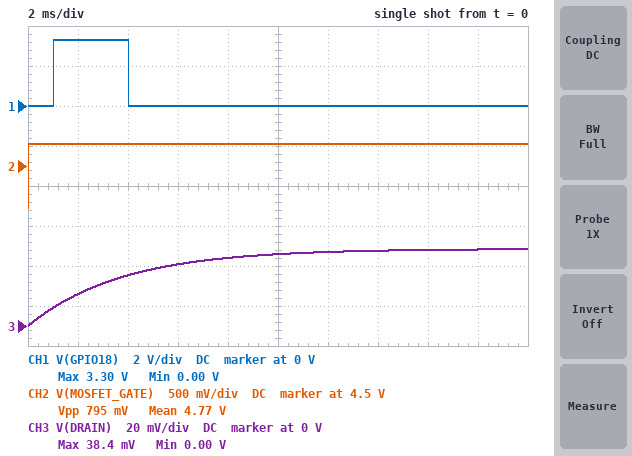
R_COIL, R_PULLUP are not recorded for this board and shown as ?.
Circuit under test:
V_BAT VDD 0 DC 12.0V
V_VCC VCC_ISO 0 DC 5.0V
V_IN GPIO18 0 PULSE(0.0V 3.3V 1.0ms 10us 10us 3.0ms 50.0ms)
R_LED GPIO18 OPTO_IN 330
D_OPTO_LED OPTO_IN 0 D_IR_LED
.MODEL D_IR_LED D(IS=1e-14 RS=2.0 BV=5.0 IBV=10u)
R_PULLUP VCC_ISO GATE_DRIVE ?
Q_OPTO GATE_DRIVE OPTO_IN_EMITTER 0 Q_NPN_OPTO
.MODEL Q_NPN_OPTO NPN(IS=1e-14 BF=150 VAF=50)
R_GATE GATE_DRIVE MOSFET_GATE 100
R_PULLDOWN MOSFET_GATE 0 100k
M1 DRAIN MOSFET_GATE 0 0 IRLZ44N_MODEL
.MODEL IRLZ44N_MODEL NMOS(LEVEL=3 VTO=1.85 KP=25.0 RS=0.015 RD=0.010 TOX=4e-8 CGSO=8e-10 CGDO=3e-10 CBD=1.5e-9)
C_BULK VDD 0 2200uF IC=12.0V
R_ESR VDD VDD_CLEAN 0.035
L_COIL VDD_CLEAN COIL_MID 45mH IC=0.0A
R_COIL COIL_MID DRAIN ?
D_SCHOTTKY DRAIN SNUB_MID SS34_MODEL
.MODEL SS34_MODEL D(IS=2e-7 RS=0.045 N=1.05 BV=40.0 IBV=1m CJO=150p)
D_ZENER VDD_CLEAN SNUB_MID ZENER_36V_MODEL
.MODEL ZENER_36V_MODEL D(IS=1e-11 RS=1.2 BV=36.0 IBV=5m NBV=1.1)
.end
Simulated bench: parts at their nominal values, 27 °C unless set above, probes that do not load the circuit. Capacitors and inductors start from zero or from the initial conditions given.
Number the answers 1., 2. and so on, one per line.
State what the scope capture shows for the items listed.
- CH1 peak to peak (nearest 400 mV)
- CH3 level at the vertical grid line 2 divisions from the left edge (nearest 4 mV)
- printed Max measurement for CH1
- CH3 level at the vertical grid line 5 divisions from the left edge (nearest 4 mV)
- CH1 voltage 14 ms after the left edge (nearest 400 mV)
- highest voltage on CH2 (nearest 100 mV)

1. 3.2 V
2. 24 mV
3. 3.30 V
4. 36 mV
5. 0 V
6. 4.8 V
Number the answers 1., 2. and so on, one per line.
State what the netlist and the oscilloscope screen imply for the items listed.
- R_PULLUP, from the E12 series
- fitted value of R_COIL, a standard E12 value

1. 4.7 kΩ
2. 12 Ω
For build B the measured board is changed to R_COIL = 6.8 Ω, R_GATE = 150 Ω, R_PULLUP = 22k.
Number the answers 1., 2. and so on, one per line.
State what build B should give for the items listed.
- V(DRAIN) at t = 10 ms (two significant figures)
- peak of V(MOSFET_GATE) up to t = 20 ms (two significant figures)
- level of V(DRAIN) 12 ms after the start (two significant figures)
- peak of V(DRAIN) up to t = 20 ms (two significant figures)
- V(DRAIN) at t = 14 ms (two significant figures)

1. 59 mV
2. 4.1 V
3. 63 mV
4. 72 mV
5. 66 mV
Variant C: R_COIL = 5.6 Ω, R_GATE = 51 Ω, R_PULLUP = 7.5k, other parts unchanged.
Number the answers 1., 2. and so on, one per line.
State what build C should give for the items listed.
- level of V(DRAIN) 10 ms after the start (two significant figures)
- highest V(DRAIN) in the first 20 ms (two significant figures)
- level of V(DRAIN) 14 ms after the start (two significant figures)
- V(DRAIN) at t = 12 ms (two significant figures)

1. 60 mV
2. 77 mV
3. 69 mV
4. 65 mV
